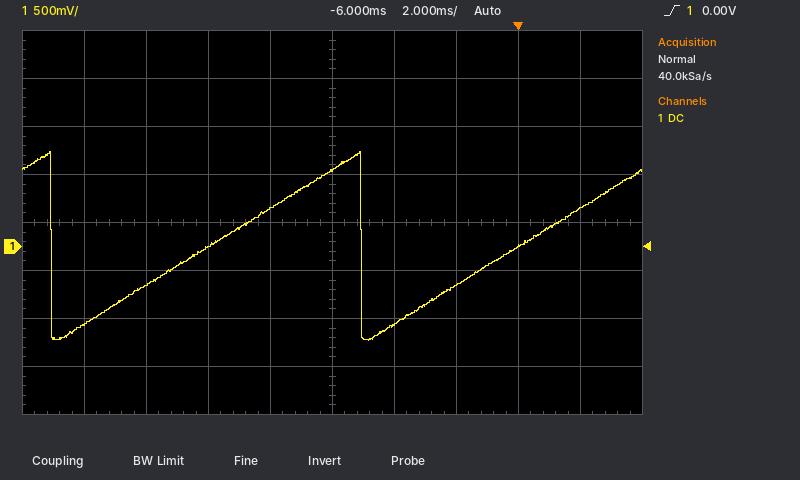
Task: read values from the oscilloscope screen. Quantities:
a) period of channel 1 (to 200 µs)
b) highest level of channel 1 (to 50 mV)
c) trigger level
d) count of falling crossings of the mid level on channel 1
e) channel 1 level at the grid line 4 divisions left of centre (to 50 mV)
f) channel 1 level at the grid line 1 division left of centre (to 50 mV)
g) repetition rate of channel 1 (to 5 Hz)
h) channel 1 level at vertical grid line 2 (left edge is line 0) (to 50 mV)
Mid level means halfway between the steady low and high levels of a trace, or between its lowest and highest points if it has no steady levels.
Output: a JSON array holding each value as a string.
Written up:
["10.0 ms", "1.00 V", "0.00 V", "2", "-800 mV", "400 mV", "100 Hz", "-400 mV"]
